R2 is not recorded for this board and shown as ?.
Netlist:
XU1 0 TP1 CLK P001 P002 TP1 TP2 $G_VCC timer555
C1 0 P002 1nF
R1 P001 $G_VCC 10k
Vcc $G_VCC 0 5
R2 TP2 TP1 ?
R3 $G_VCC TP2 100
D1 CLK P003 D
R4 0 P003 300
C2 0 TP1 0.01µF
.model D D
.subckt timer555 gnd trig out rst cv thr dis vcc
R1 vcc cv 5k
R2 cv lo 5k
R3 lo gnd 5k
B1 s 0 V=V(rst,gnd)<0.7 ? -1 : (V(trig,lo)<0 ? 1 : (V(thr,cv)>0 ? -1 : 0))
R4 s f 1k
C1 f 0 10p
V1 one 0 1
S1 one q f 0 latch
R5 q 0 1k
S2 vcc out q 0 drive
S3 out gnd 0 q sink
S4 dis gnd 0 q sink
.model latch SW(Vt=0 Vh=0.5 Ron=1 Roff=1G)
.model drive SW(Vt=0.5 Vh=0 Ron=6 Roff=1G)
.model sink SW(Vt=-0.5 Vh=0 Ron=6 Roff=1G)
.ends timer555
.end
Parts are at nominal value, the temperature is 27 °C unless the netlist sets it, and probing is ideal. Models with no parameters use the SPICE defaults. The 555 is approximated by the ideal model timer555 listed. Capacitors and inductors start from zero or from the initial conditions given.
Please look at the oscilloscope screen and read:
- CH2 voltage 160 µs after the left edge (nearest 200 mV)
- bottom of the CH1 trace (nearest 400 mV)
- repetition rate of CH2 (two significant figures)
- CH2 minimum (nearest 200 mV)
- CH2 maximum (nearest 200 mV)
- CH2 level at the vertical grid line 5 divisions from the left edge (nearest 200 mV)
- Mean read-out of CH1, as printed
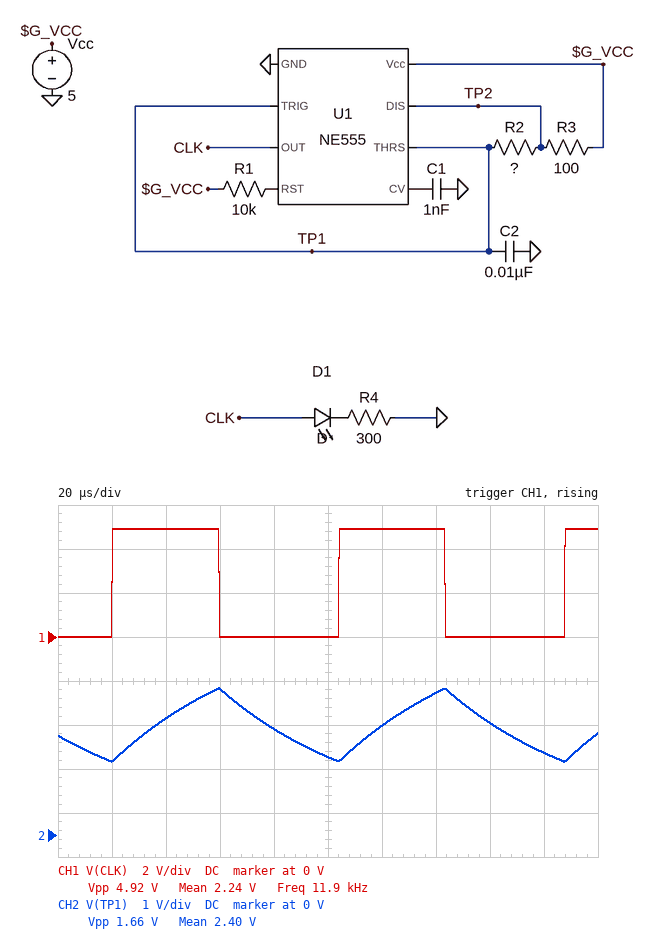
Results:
2.6 V
0 V
12 kHz
1.6 V
3.4 V
1.8 V
2.24 V
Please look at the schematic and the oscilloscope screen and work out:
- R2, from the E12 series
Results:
5.6 kΩ
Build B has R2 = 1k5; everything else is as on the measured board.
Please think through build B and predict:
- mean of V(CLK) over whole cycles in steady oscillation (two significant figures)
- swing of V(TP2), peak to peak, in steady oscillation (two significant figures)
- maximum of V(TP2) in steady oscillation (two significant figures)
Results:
2.4 V
4.6 V
4.9 V
